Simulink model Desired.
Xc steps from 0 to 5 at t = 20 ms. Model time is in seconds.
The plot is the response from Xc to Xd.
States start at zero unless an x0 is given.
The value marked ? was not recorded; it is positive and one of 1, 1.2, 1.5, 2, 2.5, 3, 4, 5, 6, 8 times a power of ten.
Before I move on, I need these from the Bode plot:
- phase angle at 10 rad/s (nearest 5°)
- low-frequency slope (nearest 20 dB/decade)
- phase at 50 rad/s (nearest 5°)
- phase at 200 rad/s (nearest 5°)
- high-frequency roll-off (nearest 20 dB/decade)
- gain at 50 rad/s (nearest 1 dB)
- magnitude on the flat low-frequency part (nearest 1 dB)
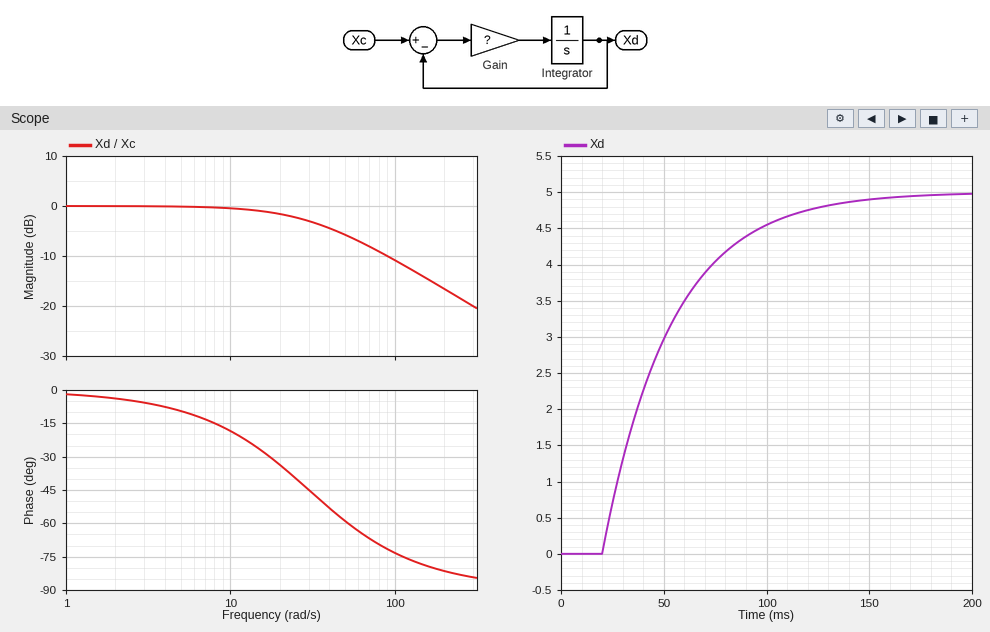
-20°
0 dB/decade
-60°
-80°
-20 dB/decade
-6 dB
0 dB
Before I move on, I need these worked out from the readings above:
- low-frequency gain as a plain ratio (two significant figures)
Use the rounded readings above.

1.0
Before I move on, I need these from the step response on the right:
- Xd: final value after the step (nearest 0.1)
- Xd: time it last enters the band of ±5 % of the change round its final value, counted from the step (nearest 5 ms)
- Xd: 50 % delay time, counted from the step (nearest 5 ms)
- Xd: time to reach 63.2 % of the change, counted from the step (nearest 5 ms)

5.0
100 ms
25 ms
35 ms
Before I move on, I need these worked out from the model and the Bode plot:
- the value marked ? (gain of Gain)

30
